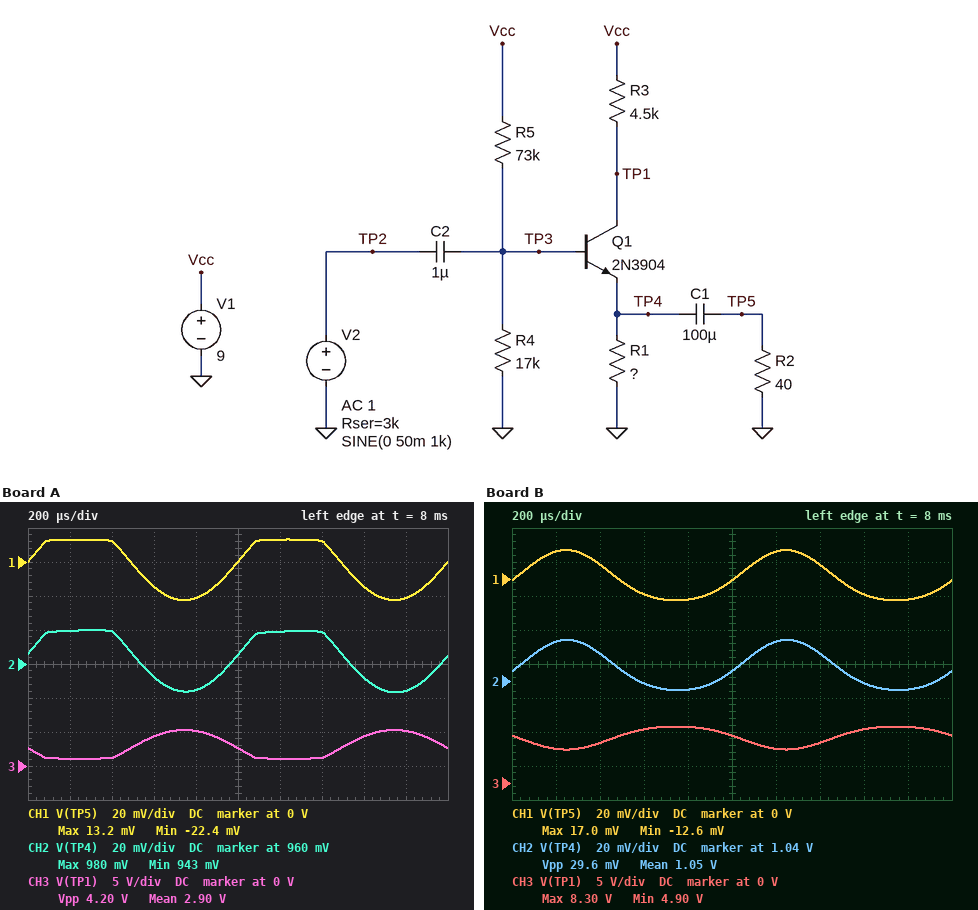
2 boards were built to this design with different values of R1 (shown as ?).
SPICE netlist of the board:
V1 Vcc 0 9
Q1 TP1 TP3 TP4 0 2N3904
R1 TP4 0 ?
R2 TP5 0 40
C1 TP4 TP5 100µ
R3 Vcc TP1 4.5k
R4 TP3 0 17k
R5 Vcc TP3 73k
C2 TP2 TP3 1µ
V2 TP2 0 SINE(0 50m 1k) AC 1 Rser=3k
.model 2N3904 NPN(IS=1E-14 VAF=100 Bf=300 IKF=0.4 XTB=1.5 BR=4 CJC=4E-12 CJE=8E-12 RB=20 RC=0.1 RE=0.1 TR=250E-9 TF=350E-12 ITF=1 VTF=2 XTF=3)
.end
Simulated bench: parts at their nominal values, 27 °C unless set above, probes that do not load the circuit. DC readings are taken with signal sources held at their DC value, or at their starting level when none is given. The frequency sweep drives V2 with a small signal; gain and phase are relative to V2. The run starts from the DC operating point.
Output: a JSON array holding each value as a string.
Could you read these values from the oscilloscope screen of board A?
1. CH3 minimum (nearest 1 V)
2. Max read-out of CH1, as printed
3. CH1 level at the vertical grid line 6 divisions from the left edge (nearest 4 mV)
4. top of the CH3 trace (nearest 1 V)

["1 V", "13.2 mV", "12 mV", "5 V"]
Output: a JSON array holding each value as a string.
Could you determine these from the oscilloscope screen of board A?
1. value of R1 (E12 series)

["680 Ω"]
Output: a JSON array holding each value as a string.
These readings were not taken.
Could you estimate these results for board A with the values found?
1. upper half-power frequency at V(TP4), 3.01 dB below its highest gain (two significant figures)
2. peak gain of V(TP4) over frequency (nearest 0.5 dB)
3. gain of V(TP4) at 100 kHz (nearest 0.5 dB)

["220 kHz", "-5.5 dB", "-7.0 dB"]
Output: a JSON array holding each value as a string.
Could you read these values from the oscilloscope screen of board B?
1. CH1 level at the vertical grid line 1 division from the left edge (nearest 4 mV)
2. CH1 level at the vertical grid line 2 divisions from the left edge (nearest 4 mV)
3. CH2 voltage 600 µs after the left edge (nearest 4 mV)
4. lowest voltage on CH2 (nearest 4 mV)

["16 mV", "8 mV", "1.040 V", "1.036 V"]
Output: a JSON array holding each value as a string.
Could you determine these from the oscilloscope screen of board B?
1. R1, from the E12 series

["2.2 kΩ"]
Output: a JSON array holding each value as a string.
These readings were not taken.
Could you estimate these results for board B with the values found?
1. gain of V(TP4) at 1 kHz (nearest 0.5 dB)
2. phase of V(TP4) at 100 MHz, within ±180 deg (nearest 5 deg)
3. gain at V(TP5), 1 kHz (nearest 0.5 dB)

["-10.0 dB", "-5 deg", "-10.0 dB"]
